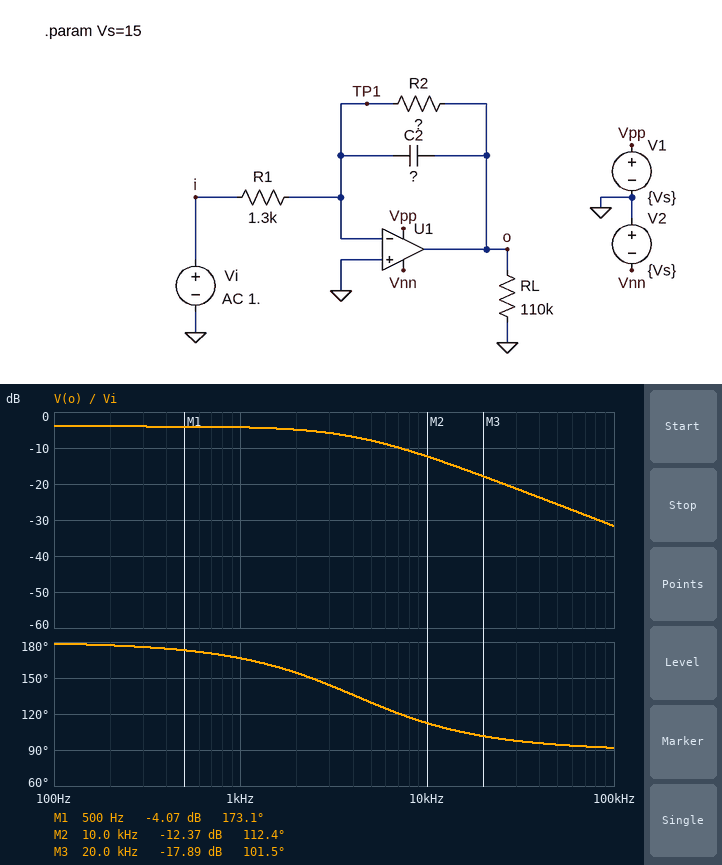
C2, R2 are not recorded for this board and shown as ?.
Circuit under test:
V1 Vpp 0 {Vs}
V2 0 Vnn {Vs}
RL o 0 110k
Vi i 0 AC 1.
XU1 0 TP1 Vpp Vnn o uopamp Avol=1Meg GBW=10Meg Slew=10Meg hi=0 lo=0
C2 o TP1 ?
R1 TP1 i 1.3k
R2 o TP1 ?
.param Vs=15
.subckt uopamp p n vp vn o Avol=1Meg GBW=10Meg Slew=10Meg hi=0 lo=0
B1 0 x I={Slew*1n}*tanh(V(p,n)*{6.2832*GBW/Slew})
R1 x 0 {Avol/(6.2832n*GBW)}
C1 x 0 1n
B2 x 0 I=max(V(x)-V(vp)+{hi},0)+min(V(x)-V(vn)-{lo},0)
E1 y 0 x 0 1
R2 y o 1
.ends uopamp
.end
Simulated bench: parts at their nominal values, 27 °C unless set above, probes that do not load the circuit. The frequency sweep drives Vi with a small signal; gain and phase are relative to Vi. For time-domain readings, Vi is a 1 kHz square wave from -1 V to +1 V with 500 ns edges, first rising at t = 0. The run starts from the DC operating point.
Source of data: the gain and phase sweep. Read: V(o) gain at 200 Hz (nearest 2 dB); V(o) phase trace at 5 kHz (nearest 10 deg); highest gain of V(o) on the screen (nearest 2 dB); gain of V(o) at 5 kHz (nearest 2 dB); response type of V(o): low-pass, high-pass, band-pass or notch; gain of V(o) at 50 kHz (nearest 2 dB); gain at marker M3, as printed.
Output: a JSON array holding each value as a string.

["-4 dB", "130 deg", "-4 dB", "-8 dB", "low-pass", "-26 dB", "-17.89 dB"]
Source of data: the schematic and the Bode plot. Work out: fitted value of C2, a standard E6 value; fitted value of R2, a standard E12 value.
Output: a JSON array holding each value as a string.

["47 nF", "820 Ω"]
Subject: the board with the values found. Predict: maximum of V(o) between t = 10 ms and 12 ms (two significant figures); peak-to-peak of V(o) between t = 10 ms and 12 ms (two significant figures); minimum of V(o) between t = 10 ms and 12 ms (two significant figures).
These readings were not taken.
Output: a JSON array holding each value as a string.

["630 mV", "1.3 V", "-630 mV"]
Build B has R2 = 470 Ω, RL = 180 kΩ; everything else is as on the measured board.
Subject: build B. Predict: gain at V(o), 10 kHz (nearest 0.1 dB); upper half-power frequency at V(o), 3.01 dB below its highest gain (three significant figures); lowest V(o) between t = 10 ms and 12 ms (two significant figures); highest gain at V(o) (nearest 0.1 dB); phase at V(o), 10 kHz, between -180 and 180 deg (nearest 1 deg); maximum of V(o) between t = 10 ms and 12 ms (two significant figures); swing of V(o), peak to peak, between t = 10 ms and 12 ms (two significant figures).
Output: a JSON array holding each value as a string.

["-13.5 dB", "7.20 kHz", "-360 mV", "-8.8 dB", "126 deg", "360 mV", "720 mV"]
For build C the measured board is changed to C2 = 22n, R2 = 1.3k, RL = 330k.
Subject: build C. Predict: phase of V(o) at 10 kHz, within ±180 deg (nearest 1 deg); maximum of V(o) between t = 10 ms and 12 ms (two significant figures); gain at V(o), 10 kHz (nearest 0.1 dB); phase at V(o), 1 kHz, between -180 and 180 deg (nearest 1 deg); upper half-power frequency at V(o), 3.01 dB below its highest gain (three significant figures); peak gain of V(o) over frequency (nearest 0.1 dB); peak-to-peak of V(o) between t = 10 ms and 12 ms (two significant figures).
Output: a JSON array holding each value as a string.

["119 deg", "1.0 V", "-6.3 dB", "170 deg", "5.56 kHz", "0 dB", "2.0 V"]
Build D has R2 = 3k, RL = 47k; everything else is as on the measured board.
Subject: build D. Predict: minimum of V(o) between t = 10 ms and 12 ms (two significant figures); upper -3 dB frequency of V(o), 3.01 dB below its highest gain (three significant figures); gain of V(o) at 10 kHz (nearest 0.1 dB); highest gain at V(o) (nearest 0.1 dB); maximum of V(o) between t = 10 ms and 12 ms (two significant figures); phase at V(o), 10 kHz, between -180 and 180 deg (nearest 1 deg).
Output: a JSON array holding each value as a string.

["-2.2 V", "1.13 kHz", "-11.7 dB", "7.3 dB", "2.2 V", "96 deg"]
